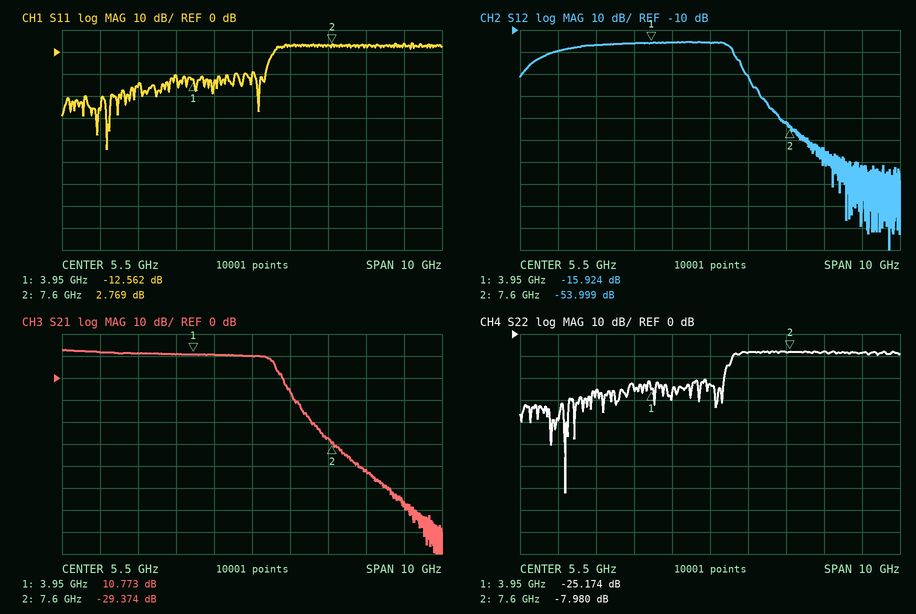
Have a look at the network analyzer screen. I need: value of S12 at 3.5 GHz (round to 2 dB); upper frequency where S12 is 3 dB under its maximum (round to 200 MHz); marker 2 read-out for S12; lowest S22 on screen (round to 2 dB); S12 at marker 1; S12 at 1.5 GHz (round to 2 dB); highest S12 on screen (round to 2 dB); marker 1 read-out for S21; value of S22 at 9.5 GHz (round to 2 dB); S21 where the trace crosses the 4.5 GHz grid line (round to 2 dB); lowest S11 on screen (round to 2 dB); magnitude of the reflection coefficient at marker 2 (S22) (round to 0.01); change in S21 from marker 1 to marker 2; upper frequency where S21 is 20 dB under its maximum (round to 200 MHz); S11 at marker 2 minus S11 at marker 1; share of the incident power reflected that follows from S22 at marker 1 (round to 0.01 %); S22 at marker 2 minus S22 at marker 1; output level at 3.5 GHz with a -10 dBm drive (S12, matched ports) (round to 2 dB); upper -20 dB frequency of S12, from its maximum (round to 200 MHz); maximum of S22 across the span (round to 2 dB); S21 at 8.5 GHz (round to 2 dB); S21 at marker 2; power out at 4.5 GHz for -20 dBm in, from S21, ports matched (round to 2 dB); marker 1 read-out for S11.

-16 dB
6.0 GHz
-53.999 dB
-72 dB
-15.924 dB
-20 dB
-16 dB
10.773 dB
-8 dB
10 dB
-44 dB
0.40
-40.147 dB
6.6 GHz
15.331 dB
0.30 %
17.194 dB
-26 dBm
6.6 GHz
-8 dB
-42 dB
-29.374 dB
-10 dBm
-12.562 dB
